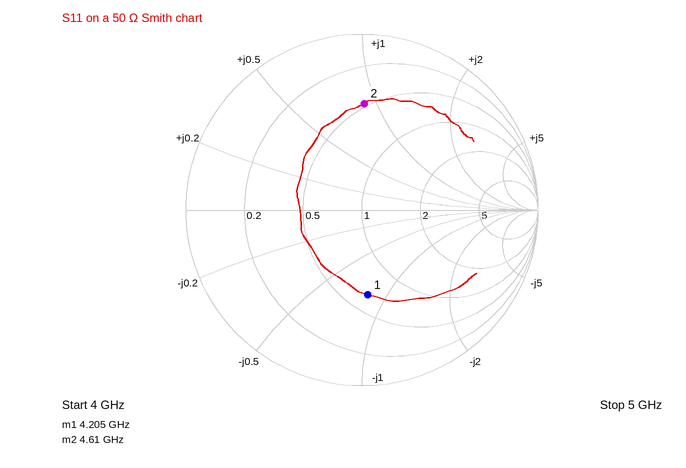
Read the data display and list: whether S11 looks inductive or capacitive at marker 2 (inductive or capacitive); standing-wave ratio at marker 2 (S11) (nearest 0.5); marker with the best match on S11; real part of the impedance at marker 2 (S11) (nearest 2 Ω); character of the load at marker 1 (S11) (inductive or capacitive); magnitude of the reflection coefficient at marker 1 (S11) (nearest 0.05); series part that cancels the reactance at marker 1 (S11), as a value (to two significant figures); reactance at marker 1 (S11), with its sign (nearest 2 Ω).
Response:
inductive
4.0
marker 1
24 Ω
capacitive
0.50
1.6 nH
-42 Ω
